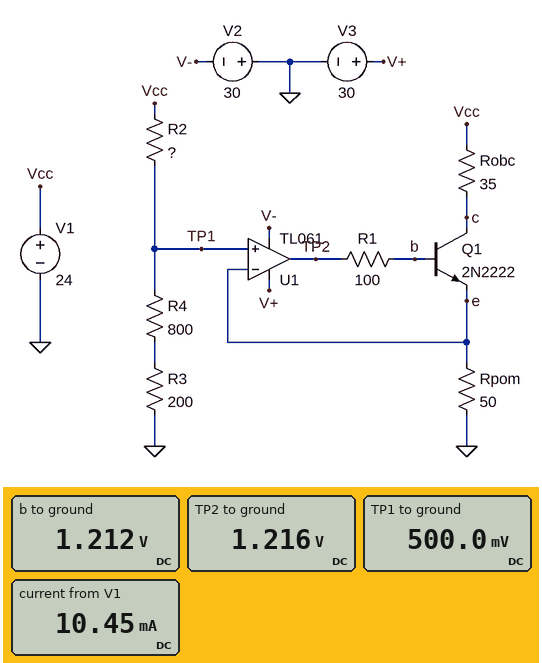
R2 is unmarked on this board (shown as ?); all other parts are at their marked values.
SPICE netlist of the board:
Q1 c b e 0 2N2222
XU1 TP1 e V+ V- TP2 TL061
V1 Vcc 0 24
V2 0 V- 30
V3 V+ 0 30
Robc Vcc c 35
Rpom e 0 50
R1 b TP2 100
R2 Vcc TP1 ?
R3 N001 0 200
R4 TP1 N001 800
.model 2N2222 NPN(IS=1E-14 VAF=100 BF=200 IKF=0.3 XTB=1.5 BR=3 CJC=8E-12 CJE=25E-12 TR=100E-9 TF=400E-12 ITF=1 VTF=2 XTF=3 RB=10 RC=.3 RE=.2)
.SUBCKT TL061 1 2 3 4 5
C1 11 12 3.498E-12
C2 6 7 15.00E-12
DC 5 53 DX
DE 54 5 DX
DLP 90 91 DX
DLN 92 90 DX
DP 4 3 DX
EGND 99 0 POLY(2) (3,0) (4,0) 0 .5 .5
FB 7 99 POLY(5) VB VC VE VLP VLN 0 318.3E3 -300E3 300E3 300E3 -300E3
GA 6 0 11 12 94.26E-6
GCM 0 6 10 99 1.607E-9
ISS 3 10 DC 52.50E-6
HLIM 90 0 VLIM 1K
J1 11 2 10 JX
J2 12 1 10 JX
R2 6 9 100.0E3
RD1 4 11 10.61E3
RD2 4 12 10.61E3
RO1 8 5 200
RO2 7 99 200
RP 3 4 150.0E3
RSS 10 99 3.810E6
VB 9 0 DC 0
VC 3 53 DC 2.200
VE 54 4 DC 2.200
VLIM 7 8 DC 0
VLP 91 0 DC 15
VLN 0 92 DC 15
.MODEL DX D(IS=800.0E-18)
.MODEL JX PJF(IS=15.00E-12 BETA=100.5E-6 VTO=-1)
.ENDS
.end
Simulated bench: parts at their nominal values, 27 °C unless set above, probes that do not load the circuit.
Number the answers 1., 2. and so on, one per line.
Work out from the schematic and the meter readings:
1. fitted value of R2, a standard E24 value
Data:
1. 47 kΩ
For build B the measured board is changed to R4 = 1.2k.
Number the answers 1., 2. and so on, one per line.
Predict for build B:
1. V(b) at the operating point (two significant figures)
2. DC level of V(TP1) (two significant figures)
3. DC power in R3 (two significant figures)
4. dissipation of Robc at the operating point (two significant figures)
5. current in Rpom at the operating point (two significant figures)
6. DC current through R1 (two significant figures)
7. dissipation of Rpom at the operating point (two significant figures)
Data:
1. 1.4 V
2. 690 mV
3. 49 µW
4. 6.7 mW
5. 14 mA
6. 59 µA
7. 9.6 mW
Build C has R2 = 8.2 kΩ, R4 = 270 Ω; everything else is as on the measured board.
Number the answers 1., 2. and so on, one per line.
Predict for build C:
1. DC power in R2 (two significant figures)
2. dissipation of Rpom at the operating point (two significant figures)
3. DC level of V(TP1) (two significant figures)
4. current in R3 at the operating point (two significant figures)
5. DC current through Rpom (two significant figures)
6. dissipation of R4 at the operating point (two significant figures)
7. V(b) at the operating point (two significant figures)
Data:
1. 63 mW
2. 34 mW
3. 1.3 V
4. 2.8 mA
5. 26 mA
6. 2.1 mW
7. 2.0 V
